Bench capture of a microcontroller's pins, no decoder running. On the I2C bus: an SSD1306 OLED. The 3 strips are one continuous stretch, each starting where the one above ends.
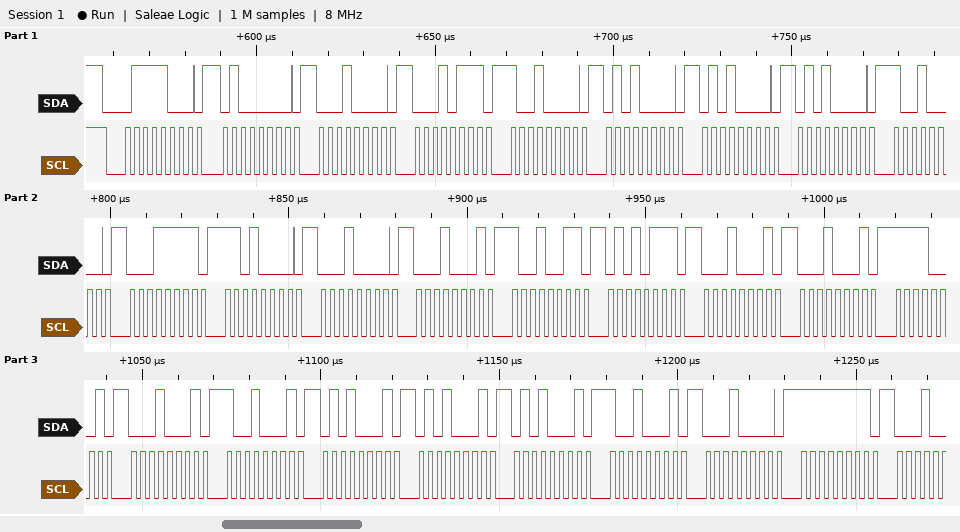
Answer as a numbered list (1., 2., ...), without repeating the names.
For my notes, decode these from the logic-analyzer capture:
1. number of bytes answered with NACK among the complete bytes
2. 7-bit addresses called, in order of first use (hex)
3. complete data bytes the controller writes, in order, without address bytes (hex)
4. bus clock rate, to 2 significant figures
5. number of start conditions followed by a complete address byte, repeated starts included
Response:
1. 0
2. 0x3C
3. 40 10 17 90 50 50 50 90 1F D0 10 11 93 57 11 11 F1 11 91 51 51 51 91 10 FF
4. 400 kHz
5. 1
